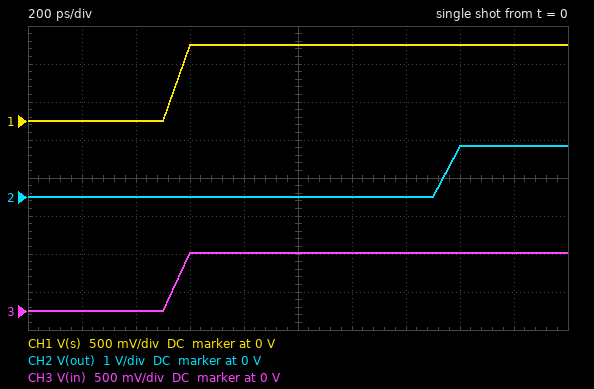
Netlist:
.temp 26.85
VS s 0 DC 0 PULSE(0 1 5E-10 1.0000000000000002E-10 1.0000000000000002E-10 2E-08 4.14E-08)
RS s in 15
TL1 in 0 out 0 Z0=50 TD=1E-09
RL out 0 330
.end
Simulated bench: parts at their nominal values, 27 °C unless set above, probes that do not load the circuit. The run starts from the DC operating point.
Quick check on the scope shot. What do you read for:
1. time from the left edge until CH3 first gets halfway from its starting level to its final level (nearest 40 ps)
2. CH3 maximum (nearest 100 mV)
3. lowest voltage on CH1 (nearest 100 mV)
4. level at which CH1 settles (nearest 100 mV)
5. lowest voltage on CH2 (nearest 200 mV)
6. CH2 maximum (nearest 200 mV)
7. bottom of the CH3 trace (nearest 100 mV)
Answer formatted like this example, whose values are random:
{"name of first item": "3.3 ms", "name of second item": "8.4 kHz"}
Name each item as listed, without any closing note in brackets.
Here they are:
{"time from the left edge until CH3 first gets halfway from its starting level to its final level": "560 ps", "CH3 maximum": "800 mV", "lowest voltage on CH1": "0 V", "level at which CH1 settles": "1.0 V", "lowest voltage on CH2": "0 V", "CH2 maximum": "1.4 V", "bottom of the CH3 trace": "0 V"}
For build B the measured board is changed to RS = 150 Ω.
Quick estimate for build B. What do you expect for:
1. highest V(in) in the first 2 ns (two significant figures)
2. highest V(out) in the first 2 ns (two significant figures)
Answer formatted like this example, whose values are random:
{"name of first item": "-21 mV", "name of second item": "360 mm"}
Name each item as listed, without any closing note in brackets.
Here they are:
{"highest V(in) in the first 2 ns": "250 mV", "highest V(out) in the first 2 ns": "430 mV"}
